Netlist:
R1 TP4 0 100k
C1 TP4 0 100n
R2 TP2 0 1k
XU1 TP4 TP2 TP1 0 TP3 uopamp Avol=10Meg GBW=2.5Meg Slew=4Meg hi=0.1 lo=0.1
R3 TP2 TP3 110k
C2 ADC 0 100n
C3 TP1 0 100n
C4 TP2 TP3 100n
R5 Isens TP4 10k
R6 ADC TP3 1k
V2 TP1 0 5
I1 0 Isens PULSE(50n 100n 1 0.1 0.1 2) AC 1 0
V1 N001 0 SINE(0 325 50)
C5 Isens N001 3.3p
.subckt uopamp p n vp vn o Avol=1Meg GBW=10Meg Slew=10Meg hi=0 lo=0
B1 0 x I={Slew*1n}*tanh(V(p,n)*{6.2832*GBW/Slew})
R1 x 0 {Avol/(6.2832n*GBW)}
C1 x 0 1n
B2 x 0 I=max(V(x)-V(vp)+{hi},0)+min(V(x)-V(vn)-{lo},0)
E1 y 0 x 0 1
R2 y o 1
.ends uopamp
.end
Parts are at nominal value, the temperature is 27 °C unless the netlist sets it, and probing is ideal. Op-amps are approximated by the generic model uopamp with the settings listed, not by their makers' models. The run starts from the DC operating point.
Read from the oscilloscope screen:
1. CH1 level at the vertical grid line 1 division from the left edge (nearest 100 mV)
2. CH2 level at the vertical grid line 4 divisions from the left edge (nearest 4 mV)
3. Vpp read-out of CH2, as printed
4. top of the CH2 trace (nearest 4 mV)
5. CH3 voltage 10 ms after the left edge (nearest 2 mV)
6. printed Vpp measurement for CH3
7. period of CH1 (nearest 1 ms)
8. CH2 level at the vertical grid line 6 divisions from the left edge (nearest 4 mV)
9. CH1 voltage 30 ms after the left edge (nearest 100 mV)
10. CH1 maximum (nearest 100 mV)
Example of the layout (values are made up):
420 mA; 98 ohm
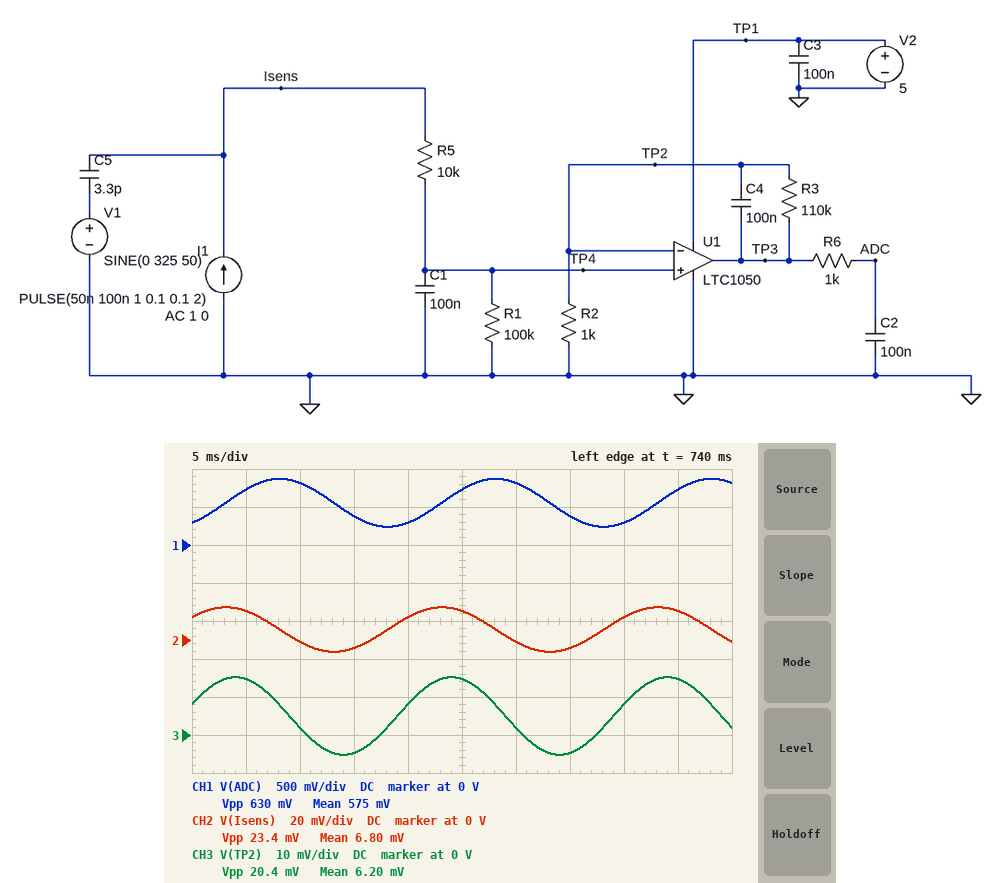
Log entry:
700 mV; 12 mV; 23.4 mV; 16 mV; 2 mV; 20.4 mV; 20 ms; 0 V; 800 mV; 900 mV
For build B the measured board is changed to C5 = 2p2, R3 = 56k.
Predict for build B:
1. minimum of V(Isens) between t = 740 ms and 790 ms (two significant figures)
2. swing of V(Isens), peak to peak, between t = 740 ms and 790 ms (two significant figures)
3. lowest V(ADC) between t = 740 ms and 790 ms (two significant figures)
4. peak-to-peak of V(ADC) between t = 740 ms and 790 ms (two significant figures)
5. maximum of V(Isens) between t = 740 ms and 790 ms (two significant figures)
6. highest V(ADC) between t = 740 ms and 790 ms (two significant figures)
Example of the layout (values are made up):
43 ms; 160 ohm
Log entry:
-2.3 mV; 16 mV; 100 mV; 380 mV; 13 mV; 480 mV
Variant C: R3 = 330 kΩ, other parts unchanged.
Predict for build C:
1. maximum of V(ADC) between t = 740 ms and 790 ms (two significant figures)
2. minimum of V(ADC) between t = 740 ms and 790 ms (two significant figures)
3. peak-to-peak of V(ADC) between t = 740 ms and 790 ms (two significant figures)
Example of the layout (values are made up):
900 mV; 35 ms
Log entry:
2.0 V; 1.3 V; 650 mV
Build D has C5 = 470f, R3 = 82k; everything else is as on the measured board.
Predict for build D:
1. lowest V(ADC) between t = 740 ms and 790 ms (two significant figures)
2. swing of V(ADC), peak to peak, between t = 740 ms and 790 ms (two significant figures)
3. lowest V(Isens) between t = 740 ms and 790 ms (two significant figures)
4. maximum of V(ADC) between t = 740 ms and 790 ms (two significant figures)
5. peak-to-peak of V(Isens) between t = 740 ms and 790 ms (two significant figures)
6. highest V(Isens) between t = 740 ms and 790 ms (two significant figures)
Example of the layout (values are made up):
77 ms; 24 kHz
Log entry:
370 mV; 87 mV; 3.8 mV; 460 mV; 3.3 mV; 7.2 mV
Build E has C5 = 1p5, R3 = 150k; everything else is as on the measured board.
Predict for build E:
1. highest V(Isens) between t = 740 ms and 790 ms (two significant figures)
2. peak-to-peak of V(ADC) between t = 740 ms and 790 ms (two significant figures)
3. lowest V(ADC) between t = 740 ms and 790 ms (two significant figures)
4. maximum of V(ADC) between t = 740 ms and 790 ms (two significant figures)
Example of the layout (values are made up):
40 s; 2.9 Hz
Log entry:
11 mV; 290 mV; 610 mV; 900 mV
